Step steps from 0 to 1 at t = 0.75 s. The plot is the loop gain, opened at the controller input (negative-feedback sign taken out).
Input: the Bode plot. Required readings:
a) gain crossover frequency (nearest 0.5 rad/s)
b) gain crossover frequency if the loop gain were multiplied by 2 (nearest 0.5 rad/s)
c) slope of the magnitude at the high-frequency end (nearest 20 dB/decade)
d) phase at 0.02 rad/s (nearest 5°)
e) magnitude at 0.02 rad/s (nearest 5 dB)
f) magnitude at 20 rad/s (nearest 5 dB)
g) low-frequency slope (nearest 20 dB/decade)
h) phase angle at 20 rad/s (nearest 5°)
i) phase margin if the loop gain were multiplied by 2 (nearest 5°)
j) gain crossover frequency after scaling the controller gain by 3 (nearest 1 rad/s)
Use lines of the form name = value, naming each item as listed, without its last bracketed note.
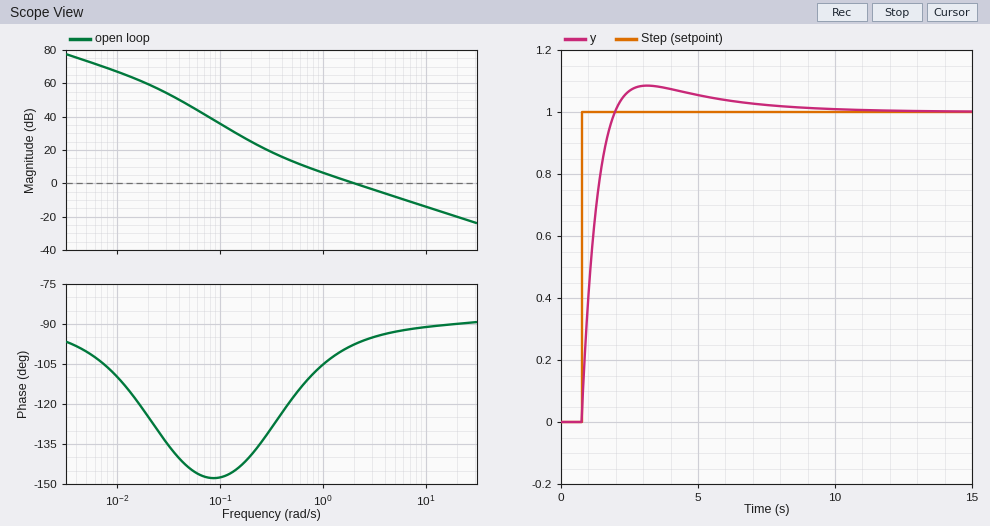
gain crossover frequency = 2.0 rad/s
gain crossover frequency if the loop gain were multiplied by 2 = 4.0 rad/s
slope of the magnitude at the high-frequency end = -20 dB/decade
phase at 0.02 rad/s = -125°
magnitude at 0.02 rad/s = 60 dB
magnitude at 20 rad/s = -20 dB
low-frequency slope = -20 dB/decade
phase angle at 20 rad/s = -90°
phase margin if the loop gain were multiplied by 2 = 85°
gain crossover frequency after scaling the controller gain by 3 = 6 rad/s
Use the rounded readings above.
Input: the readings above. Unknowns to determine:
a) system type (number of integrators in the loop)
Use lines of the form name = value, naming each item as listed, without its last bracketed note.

system type = 1
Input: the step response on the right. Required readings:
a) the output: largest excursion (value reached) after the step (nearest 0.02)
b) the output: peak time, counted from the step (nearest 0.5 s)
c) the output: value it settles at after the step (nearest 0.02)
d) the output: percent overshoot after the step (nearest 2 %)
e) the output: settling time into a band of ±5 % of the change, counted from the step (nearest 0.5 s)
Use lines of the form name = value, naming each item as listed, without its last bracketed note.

the output: largest excursion (value reached) after the step = 1.08
the output: peak time, counted from the step = 2.5 s
the output: value it settles at after the step = 1.00
the output: percent overshoot after the step = 8 %
the output: settling time into a band of ±5 % of the change, counted from the step = 4.5 s
